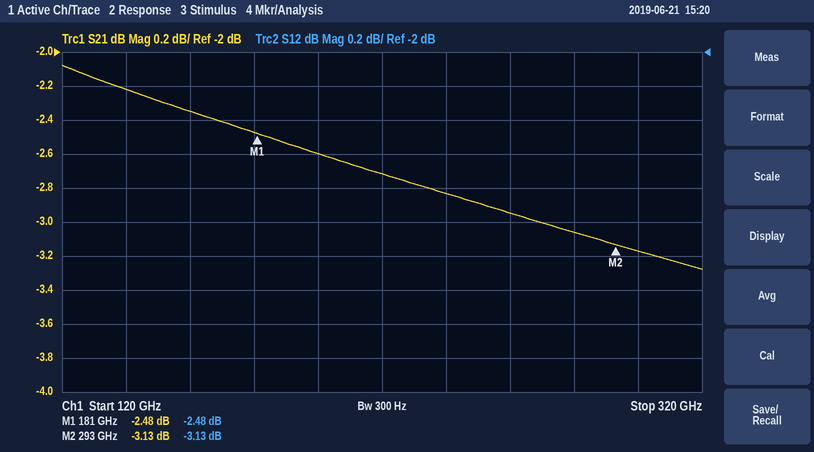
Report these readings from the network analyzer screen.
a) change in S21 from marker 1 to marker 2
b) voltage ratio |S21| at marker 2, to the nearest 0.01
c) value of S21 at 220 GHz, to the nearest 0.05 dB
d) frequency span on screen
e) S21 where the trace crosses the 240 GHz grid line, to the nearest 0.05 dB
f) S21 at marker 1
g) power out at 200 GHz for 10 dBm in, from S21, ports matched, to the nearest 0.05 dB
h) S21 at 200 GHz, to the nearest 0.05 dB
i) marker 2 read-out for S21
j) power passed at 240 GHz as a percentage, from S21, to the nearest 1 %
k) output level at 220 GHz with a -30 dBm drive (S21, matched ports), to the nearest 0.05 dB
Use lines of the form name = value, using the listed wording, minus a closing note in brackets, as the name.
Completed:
change in S21 from marker 1 to marker 2 = -0.65 dB
voltage ratio |S21| at marker 2, to the nearest 0.01 = 0.70
value of S21 at 220 GHz, to the nearest 0.05 dB = -2.70 dB
frequency span on screen = 200 GHz
S21 where the trace crosses the 240 GHz grid line, to the nearest 0.05 dB = -2.85 dB
S21 at marker 1 = -2.48 dB
power out at 200 GHz for 10 dBm in, from S21, ports matched, to the nearest 0.05 dB = 7.40 dBm
S21 at 200 GHz, to the nearest 0.05 dB = -2.60 dB
marker 2 read-out for S21 = -3.13 dB
power passed at 240 GHz as a percentage, from S21, to the nearest 1 % = 52 %
output level at 220 GHz with a -30 dBm drive (S21, matched ports), to the nearest 0.05 dB = -32.70 dBm
